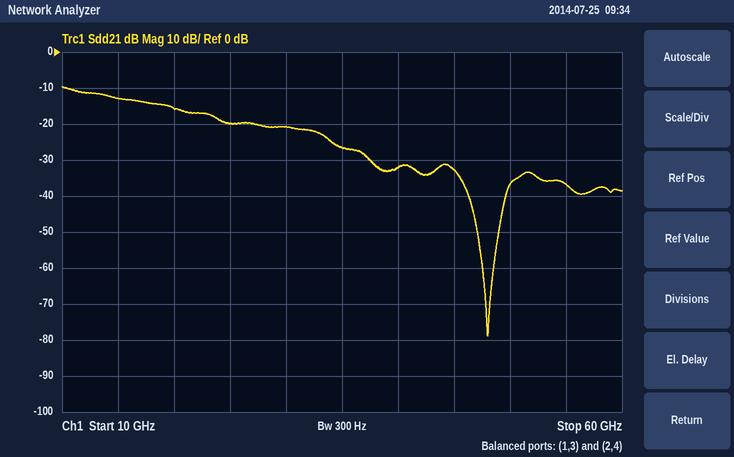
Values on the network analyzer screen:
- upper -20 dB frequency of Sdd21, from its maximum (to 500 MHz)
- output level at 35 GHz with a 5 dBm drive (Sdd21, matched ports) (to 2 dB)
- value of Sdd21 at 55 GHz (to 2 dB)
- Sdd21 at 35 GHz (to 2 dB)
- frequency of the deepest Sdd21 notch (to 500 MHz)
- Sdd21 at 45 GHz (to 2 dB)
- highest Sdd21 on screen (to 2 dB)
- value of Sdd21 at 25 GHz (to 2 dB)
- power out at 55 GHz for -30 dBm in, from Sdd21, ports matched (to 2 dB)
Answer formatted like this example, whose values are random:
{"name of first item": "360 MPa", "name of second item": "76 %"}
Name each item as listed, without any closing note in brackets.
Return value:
{"upper -20 dB frequency of Sdd21, from its maximum": "37.5 GHz", "output level at 35 GHz with a 5 dBm drive (Sdd21, matched ports)": "-22 dBm", "value of Sdd21 at 55 GHz": "-36 dB", "Sdd21 at 35 GHz": "-26 dB", "frequency of the deepest Sdd21 notch": "48.0 GHz", "Sdd21 at 45 GHz": "-32 dB", "highest Sdd21 on screen": "-10 dB", "value of Sdd21 at 25 GHz": "-20 dB", "power out at 55 GHz for -30 dBm in, from Sdd21, ports matched": "-66 dBm"}
